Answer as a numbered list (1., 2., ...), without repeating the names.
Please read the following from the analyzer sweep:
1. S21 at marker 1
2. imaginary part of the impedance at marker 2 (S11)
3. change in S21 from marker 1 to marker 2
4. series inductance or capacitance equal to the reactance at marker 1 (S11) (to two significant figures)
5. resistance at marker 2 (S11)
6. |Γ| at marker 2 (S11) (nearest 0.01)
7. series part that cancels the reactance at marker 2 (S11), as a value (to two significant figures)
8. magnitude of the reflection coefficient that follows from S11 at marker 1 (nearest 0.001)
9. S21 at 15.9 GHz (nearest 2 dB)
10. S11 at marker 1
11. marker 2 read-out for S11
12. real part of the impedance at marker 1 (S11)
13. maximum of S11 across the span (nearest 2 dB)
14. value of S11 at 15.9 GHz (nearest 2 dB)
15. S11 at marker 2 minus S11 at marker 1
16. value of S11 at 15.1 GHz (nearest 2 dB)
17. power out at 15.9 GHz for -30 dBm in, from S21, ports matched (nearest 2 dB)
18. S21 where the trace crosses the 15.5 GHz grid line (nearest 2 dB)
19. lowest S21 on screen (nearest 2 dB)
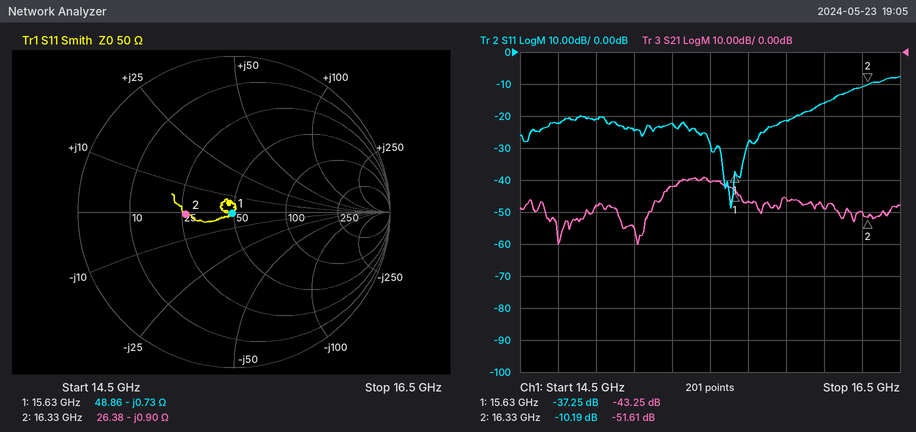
1. -43.25 dB
2. -0.90 Ω
3. -8.36 dB
4. 14 pF
5. 26.38 Ω
6. 0.31
7. 8.8 pH
8. 0.014
9. -46 dB
10. -37.25 dB
11. -10.19 dB
12. 48.86 Ω
13. -8 dB
14. -22 dB
15. 27.06 dB
16. -24 dB
17. -76 dBm
18. -40 dB
19. -60 dB
